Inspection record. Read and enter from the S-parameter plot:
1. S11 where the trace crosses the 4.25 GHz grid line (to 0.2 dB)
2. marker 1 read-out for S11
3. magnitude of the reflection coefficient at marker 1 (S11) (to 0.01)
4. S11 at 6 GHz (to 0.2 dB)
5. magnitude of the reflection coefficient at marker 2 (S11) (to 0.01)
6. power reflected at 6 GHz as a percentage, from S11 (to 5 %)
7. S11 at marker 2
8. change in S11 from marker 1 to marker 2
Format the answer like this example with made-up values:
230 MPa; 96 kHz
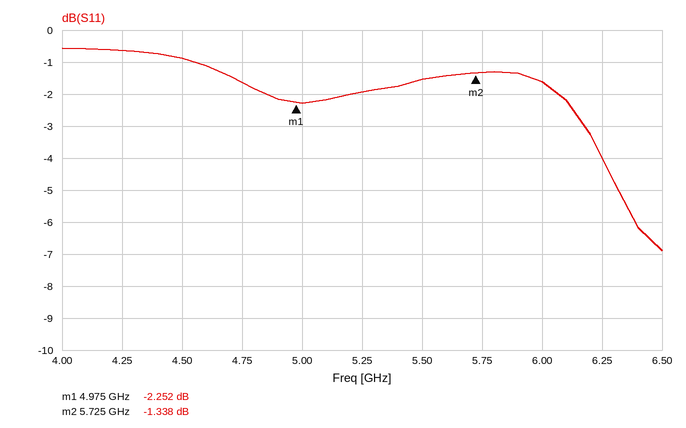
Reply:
-0.6 dB; -2.252 dB; 0.77; -1.6 dB; 0.86; 70 %; -1.338 dB; 0.914 dB
